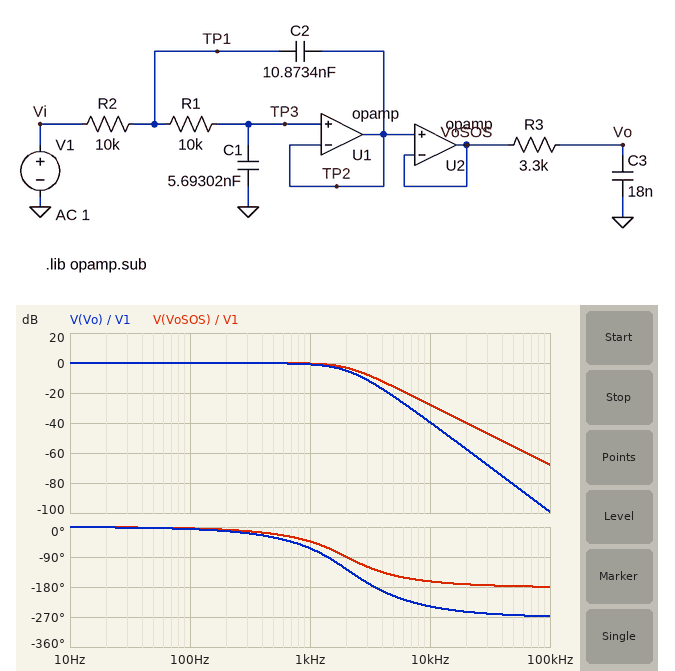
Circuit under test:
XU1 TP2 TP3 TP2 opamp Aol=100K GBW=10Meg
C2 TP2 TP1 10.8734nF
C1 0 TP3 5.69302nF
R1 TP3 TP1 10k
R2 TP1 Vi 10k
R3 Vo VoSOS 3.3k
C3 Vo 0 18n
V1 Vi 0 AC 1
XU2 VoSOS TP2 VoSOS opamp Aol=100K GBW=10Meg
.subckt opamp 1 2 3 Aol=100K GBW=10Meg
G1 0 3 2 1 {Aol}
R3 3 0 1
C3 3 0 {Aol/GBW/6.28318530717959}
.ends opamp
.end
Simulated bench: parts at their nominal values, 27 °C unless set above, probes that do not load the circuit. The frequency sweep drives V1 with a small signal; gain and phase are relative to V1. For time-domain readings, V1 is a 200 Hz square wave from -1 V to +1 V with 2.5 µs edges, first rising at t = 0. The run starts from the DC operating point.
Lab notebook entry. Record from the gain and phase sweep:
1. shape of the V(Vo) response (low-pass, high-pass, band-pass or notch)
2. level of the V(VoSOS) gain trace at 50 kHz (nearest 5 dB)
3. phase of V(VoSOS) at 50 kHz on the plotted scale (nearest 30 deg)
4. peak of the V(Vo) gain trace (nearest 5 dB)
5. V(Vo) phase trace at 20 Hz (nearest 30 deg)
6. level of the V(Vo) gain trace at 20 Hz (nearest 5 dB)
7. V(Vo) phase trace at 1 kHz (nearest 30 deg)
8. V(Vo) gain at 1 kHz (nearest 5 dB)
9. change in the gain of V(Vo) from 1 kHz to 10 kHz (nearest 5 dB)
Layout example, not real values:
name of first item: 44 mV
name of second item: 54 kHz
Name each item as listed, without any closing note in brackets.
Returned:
shape of the V(Vo) response: low-pass
level of the V(VoSOS) gain trace at 50 kHz: -55 dB
phase of V(VoSOS) at 50 kHz on the plotted scale: -180 deg
peak of the V(Vo) gain trace: 0 dB
V(Vo) phase trace at 20 Hz: 0 deg
level of the V(Vo) gain trace at 20 Hz: 0 dB
V(Vo) phase trace at 1 kHz: -60 deg
V(Vo) gain at 1 kHz: 0 dB
change in the gain of V(Vo) from 1 kHz to 10 kHz: -40 dB
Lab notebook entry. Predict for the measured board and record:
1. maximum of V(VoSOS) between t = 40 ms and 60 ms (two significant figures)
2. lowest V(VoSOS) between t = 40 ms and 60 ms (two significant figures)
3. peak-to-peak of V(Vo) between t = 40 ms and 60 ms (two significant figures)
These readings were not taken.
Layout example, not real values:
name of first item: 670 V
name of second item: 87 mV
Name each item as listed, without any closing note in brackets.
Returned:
maximum of V(VoSOS) between t = 40 ms and 60 ms: 1.1 V
lowest V(VoSOS) between t = 40 ms and 60 ms: -1.1 V
peak-to-peak of V(Vo) between t = 40 ms and 60 ms: 2.1 V
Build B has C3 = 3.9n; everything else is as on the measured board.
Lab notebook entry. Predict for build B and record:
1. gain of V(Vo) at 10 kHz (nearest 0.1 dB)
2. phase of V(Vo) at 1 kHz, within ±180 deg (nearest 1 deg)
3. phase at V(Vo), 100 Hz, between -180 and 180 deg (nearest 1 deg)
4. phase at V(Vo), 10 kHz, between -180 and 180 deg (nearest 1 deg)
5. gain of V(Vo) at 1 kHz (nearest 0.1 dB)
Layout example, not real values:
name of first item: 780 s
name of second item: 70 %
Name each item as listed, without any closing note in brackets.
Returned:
gain of V(Vo) at 10 kHz: -30.0 dB
phase of V(Vo) at 1 kHz, within ±180 deg: -48 deg
phase at V(Vo), 100 Hz, between -180 and 180 deg: -5 deg
phase at V(Vo), 10 kHz, between -180 and 180 deg: 158 deg
gain of V(Vo) at 1 kHz: -0.4 dB
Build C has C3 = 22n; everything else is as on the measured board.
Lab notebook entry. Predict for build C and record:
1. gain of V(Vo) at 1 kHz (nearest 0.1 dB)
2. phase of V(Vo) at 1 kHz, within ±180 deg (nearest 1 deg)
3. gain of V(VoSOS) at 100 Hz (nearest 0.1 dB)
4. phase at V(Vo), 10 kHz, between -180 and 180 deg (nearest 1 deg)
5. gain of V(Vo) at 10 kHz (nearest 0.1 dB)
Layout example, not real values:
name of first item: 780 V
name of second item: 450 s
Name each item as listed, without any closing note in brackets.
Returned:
gain of V(Vo) at 1 kHz: -1.2 dB
phase of V(Vo) at 1 kHz, within ±180 deg: -68 deg
gain of V(VoSOS) at 100 Hz: 0 dB
phase at V(Vo), 10 kHz, between -180 and 180 deg: 119 deg
gain of V(Vo) at 10 kHz: -41.2 dB
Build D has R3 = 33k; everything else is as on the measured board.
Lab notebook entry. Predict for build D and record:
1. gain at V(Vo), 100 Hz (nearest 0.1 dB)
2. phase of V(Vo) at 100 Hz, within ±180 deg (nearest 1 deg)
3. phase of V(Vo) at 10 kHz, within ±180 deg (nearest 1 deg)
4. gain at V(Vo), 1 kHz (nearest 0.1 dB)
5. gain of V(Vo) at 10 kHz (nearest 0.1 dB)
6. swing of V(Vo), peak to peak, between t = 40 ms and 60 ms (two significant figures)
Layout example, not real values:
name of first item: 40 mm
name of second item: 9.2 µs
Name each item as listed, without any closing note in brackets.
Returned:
gain at V(Vo), 100 Hz: -0.6 dB
phase of V(Vo) at 100 Hz, within ±180 deg: -25 deg
phase of V(Vo) at 10 kHz, within ±180 deg: 108 deg
gain at V(Vo), 1 kHz: -12.1 dB
gain of V(Vo) at 10 kHz: -59.2 dB
swing of V(Vo), peak to peak, between t = 40 ms and 60 ms: 1.9 V
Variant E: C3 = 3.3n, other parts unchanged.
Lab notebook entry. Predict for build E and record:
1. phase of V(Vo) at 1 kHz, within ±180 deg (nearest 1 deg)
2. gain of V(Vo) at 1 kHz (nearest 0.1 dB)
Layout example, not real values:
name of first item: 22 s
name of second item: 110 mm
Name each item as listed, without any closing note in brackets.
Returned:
phase of V(Vo) at 1 kHz, within ±180 deg: -47 deg
gain of V(Vo) at 1 kHz: -0.4 dB
